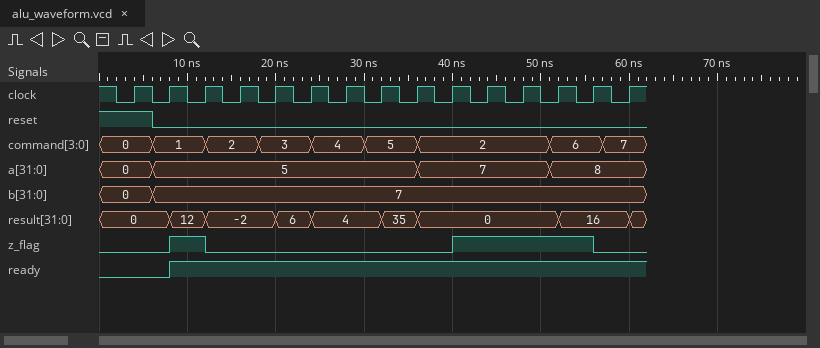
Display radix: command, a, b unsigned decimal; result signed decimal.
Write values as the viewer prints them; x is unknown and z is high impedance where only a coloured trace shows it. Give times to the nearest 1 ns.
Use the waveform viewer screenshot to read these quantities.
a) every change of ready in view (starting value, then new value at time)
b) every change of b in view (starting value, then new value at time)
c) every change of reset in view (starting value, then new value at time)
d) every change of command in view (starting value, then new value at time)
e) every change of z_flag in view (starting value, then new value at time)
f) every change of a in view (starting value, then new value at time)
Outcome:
0, 1 at 8 ns
0, 7 at 6 ns
1, 0 at 6 ns
0, 1 at 6 ns, 2 at 12 ns, 3 at 18 ns, 4 at 24 ns, 5 at 30 ns, 2 at 36 ns, 6 at 51 ns, 7 at 57 ns
0, 1 at 8 ns, 0 at 12 ns, 1 at 40 ns, 0 at 56 ns
0, 5 at 6 ns, 7 at 36 ns, 8 at 51 ns
